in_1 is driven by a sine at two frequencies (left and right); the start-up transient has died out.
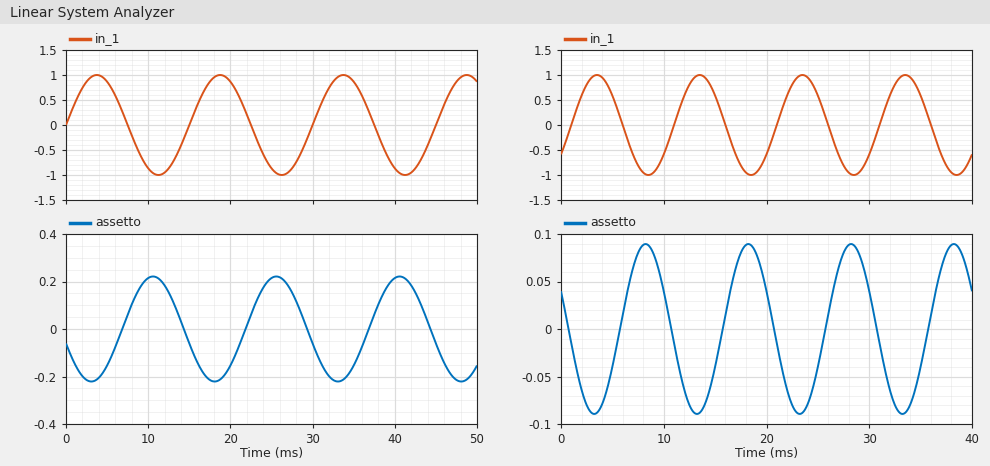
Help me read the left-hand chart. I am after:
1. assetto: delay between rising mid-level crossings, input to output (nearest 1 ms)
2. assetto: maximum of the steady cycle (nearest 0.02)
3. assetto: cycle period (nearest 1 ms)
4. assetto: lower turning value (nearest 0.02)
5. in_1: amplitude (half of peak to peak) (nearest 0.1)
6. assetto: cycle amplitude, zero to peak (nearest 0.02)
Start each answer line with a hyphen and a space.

- 7 ms
- 0.22
- 15 ms
- -0.22
- 1.0
- 0.22
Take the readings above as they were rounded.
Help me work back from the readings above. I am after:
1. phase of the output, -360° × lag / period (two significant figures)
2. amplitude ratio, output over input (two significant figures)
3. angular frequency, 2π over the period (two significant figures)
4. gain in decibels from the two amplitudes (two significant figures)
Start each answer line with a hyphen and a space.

- -170°
- 0.22
- 0.42 rad/ms
- -13 dB
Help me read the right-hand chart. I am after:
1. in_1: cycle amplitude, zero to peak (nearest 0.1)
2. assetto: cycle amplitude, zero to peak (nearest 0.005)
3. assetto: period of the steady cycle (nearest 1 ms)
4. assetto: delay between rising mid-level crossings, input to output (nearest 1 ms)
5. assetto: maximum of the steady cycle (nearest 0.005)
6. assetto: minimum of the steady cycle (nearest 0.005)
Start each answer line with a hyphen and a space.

- 1.0
- 0.090
- 10 ms
- 5 ms
- 0.090
- -0.090
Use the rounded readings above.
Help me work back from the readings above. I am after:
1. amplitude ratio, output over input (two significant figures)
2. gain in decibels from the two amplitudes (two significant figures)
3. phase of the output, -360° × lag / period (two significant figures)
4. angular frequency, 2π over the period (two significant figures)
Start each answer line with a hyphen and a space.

- 0.090
- -21 dB
- -180°
- 0.63 rad/ms
